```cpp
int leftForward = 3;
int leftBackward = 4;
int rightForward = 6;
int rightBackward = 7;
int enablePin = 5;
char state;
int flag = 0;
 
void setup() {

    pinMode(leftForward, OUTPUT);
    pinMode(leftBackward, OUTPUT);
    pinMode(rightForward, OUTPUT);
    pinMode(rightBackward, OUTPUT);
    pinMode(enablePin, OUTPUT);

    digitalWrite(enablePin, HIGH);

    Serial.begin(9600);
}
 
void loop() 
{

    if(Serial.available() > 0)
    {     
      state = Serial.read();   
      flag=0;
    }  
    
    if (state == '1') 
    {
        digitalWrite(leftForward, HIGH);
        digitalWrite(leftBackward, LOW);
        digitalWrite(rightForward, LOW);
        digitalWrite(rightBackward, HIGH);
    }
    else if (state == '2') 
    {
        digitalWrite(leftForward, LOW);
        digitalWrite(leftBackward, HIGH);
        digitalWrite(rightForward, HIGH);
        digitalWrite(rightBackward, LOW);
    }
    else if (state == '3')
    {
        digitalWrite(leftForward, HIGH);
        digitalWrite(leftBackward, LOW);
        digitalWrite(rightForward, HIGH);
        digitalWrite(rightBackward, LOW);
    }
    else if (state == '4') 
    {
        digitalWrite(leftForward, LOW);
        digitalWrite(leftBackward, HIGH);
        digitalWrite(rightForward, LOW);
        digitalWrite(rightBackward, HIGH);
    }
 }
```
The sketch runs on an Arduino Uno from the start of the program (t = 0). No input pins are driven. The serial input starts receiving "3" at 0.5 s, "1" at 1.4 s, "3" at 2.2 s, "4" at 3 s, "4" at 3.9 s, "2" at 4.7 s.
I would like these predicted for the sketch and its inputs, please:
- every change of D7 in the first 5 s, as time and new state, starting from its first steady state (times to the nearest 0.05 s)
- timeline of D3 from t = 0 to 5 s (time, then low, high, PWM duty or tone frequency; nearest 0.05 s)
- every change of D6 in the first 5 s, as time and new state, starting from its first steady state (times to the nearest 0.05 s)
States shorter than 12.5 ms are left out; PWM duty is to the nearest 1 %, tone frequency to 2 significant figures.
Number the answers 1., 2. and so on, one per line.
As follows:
1. 0 s low; 1.4 s high; 2.2 s low; 3 s high; 4.7 s low
2. 0 s low; 0.5 s high; 3 s low
3. 0 s low; 0.5 s high; 1.4 s low; 2.2 s high; 3 s low; 4.7 s high
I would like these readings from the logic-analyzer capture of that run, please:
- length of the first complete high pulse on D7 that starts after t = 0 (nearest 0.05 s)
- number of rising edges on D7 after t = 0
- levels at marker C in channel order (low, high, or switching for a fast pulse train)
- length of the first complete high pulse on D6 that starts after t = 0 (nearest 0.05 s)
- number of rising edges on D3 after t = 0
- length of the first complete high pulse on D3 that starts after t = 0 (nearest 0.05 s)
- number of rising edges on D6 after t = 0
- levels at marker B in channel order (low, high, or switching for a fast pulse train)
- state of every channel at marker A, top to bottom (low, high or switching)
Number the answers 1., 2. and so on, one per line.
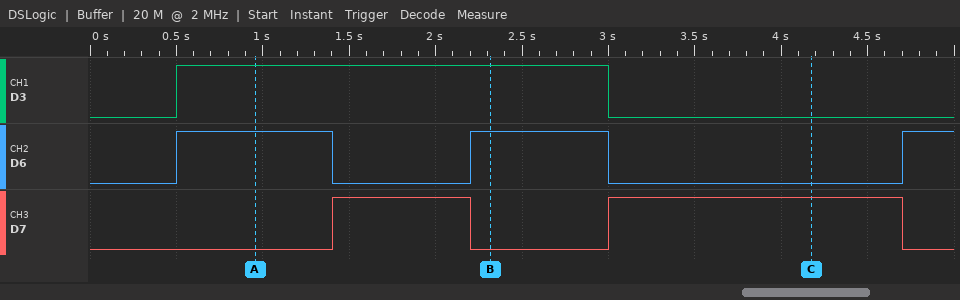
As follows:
1. 0.80 s
2. 2
3. D3 low, D6 low, D7 high
4. 0.90 s
5. 1
6. 2.50 s
7. 3
8. D3 high, D6 high, D7 low
9. D3 high, D6 high, D7 low
